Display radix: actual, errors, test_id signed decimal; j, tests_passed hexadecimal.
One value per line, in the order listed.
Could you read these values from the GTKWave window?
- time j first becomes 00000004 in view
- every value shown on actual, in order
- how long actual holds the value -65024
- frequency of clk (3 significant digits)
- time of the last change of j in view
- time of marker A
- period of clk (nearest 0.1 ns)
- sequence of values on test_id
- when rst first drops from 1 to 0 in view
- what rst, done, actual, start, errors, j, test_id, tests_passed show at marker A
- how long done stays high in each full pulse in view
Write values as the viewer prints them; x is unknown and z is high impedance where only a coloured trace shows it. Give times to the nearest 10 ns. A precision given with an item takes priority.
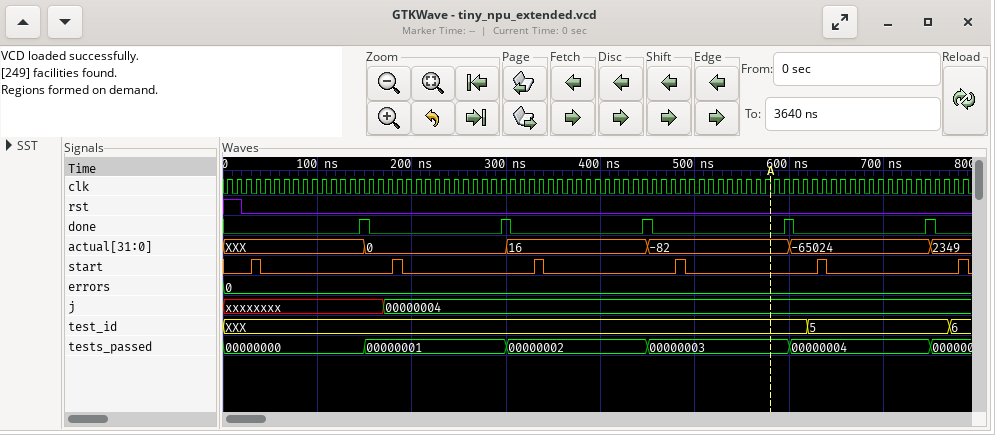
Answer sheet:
170 ns
XXX, 0, 16, -82, -65024, 2349
150 ns
100 MHz
170 ns
580 ns
10 ns
XXX, 5, 6
20 ns
rst=0, done=0, actual=-82, start=0, errors=0, j=00000004, test_id=XXX, tests_passed=00000003
10 ns, 10 ns, 10 ns, 10 ns, 10 ns
